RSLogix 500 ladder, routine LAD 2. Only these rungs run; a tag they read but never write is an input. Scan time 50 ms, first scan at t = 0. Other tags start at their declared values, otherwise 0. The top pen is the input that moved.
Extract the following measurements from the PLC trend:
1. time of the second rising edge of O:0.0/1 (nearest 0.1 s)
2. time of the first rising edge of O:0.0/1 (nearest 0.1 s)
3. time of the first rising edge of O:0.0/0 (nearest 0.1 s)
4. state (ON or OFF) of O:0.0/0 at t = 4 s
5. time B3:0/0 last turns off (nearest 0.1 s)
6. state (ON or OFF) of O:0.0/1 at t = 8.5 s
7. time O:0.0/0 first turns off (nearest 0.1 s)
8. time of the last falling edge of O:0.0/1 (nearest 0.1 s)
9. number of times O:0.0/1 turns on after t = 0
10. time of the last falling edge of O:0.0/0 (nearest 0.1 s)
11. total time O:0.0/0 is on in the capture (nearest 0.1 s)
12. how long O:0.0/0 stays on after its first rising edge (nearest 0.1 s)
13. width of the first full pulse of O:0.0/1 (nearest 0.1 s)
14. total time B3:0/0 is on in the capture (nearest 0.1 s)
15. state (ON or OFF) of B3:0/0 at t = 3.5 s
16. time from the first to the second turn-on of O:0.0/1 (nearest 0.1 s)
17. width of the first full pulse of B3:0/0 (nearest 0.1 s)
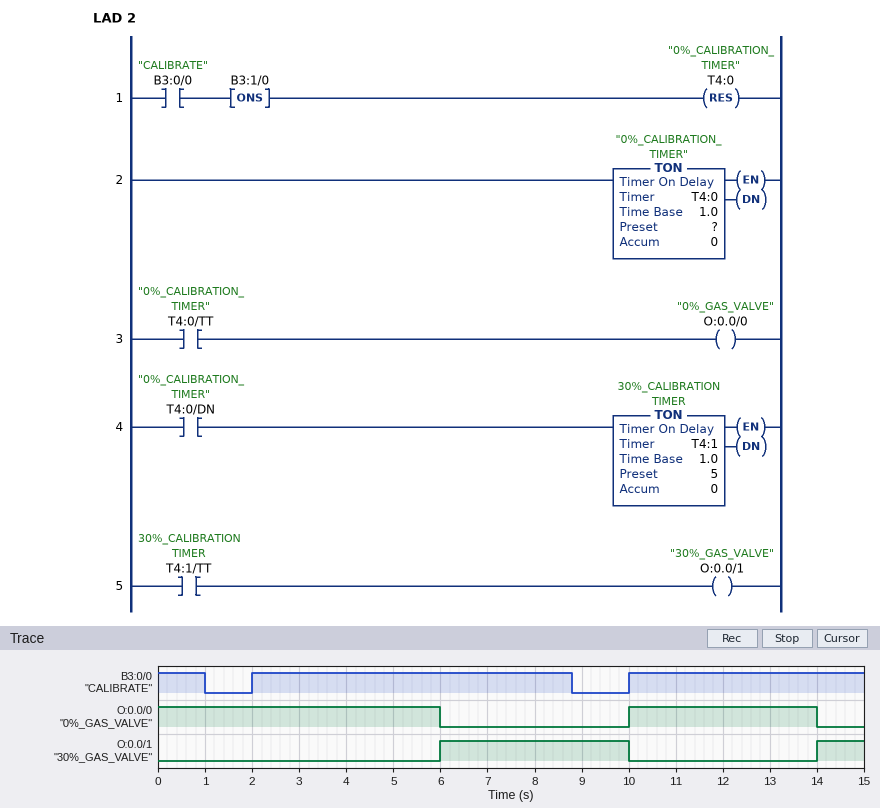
14.0 s
6.0 s
10.0 s
ON
8.8 s
ON
6.0 s
10.0 s
2
14.0 s
10.0 s
4.0 s
4.0 s
12.8 s
ON
8.0 s
6.8 s
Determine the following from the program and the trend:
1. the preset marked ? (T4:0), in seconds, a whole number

4 s
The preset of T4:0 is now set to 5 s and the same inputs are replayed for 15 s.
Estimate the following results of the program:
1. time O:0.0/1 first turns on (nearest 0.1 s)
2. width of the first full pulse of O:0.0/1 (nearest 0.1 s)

7.0 s
3.0 s
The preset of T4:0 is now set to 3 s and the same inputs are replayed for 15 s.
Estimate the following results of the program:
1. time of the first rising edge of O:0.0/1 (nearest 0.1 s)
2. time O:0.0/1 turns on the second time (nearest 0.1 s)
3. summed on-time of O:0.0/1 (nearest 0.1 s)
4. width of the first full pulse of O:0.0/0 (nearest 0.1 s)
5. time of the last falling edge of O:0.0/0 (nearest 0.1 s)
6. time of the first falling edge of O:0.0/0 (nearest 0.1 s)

5.0 s
13.0 s
7.0 s
3.0 s
13.0 s
5.0 s
